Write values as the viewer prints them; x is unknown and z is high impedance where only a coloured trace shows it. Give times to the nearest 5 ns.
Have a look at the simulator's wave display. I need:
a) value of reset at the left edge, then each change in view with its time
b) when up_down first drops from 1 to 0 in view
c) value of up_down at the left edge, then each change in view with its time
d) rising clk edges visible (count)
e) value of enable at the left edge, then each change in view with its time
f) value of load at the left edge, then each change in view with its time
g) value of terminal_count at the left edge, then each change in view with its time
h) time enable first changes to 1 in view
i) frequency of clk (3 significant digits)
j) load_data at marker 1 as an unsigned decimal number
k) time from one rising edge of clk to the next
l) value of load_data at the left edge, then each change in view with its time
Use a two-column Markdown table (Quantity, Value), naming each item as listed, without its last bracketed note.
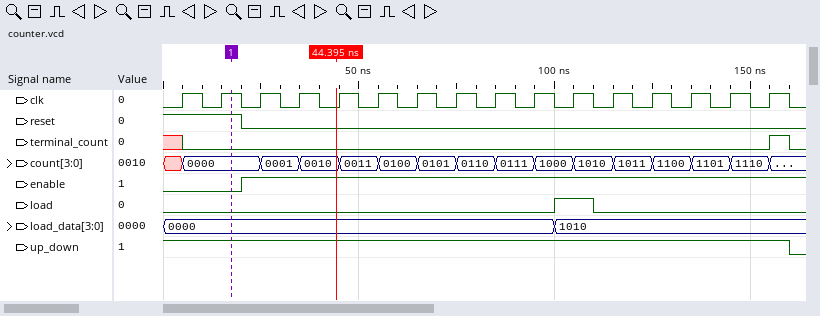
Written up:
| Quantity | Value |
|---|---|
| value of reset at the left edge, then each change in view with its time | 1, 0 at 20 ns |
| when up_down first drops from 1 to 0 in view | 160 ns |
| value of up_down at the left edge, then each change in view with its time | 1, 0 at 160 ns |
| rising clk edges visible | 16 |
| value of enable at the left edge, then each change in view with its time | 0, 1 at 20 ns |
| value of load at the left edge, then each change in view with its time | 0, 1 at 100 ns, 0 at 110 ns |
| value of terminal_count at the left edge, then each change in view with its time | x, 0 at 5 ns, 1 at 155 ns, 0 at 160 ns |
| time enable first changes to 1 in view | 20 ns |
| frequency of clk | 100 MHz |
| load_data at marker 1 as an unsigned decimal number | 0 |
| time from one rising edge of clk to the next | 10 ns |
| value of load_data at the left edge, then each change in view with its time | 0000, 1010 at 100 ns |
